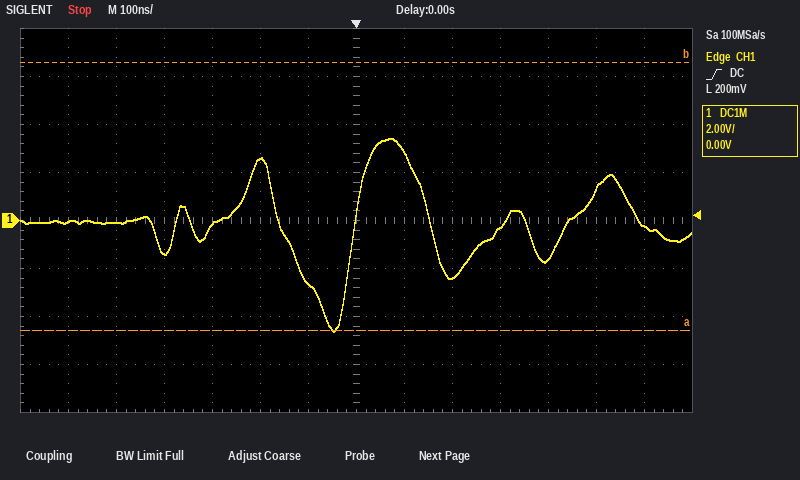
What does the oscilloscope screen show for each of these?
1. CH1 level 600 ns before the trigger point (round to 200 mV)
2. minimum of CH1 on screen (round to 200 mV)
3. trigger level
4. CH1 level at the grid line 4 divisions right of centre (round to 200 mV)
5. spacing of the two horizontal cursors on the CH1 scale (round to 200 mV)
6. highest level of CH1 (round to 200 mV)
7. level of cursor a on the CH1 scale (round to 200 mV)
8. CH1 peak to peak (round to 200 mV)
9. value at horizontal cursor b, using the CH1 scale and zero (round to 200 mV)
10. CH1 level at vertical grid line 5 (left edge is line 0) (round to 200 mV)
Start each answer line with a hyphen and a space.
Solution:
- 0.0 V
- -4.6 V
- 200 mV
- -1.6 V
- 11.2 V
- 3.4 V
- -4.6 V
- 8.0 V
- 6.6 V
- 2.6 V
